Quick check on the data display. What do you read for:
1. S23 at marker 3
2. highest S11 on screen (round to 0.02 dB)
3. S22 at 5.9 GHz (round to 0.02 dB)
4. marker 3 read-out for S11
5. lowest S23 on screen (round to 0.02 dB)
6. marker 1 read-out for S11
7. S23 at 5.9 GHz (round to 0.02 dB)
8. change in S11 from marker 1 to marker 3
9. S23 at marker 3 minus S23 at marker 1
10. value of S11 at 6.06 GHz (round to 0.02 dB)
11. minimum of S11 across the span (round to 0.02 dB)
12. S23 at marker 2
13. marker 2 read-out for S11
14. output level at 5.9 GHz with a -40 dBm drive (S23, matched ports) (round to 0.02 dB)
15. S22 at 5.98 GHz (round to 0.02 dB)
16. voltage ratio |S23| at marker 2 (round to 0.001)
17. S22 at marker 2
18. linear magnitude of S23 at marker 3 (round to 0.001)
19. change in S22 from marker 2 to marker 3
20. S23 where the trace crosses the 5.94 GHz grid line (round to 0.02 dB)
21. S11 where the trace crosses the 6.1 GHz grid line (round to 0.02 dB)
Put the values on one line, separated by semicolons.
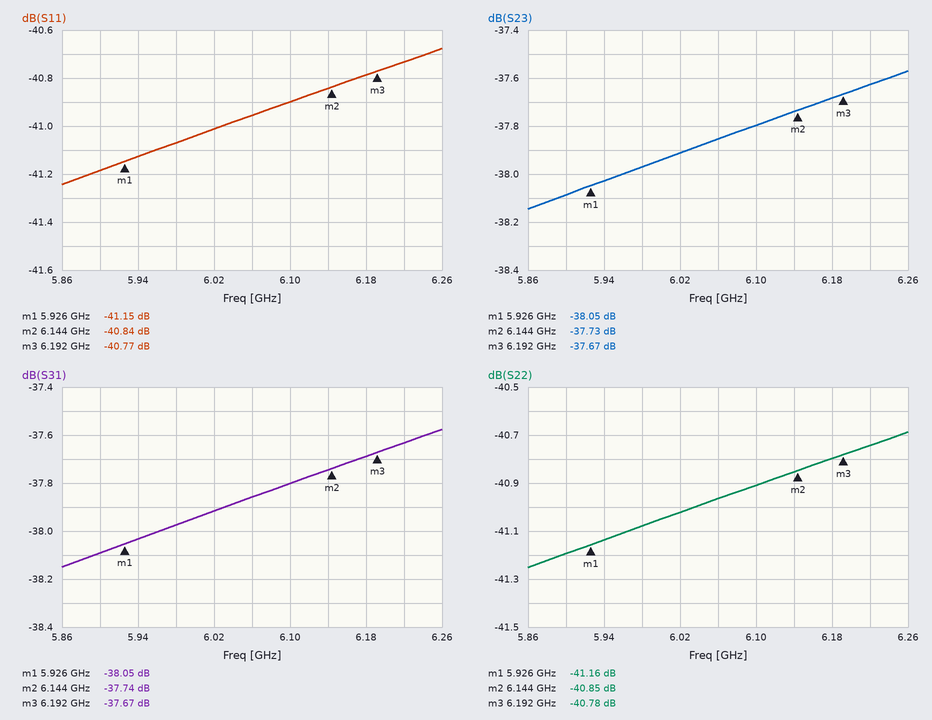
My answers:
-37.67 dB; -40.68 dB; -41.20 dB; -40.77 dB; -38.14 dB; -41.15 dB; -38.08 dB; 0.38 dB; 0.38 dB; -40.96 dB; -41.24 dB; -37.73 dB; -40.84 dB; -78.08 dBm; -41.08 dB; 0.013; -40.85 dB; 0.013; 0.07 dB; -38.02 dB; -40.90 dB
